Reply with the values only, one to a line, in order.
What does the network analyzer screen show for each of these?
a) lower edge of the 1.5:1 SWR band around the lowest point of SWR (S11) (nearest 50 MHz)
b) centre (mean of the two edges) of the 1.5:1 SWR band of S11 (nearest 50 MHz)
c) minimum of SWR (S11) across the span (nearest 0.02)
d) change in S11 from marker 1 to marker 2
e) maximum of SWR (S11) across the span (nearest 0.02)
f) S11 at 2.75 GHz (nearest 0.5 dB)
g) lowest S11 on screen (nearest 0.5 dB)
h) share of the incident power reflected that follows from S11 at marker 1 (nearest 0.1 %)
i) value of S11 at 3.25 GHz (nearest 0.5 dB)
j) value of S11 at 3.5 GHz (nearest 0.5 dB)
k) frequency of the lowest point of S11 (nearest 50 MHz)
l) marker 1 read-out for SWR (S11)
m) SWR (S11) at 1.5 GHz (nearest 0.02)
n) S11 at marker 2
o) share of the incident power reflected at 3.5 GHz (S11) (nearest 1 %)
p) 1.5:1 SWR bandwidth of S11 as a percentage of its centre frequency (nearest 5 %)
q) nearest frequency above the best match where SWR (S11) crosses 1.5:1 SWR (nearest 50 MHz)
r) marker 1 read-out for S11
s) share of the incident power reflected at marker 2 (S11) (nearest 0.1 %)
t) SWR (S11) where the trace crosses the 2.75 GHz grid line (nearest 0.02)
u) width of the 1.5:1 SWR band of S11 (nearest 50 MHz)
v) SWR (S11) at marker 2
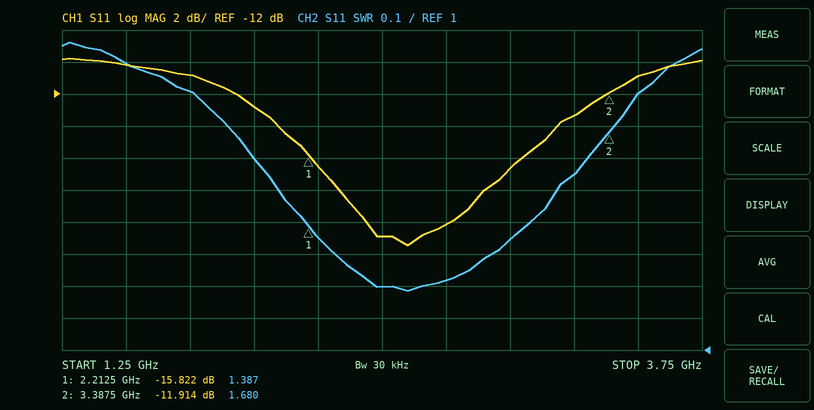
2.10 GHz
2.65 GHz
1.18
3.908 dB
1.96
-20.0 dB
-21.5 dB
2.6 %
-13.5 dB
-11.0 dB
2.60 GHz
1.387
1.90
-11.914 dB
8 %
40 %
3.20 GHz
-15.822 dB
6.4 %
1.22
1.10 GHz
1.680
